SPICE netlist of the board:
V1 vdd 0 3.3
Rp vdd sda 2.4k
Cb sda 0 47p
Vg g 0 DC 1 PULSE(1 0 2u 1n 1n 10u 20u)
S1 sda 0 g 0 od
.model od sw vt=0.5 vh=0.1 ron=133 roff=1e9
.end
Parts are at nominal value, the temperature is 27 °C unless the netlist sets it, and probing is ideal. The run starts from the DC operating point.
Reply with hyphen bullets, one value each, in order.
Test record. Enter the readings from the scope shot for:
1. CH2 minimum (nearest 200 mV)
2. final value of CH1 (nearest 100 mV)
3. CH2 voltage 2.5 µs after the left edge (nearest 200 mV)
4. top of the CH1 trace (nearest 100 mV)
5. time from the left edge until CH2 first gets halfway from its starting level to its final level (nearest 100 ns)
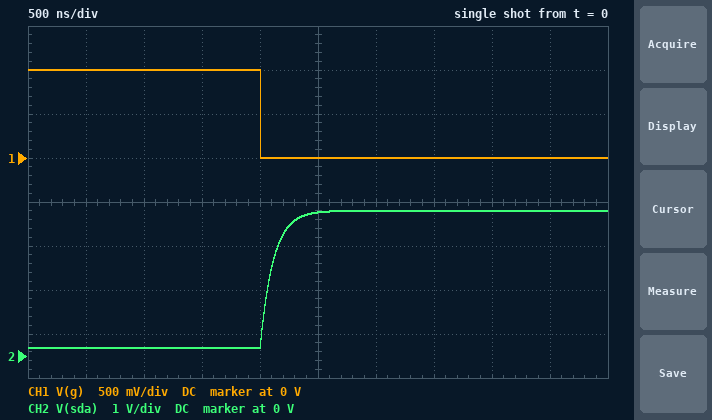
- 200 mV
- 0 V
- 3.2 V
- 1.0 V
- 2.1 µs
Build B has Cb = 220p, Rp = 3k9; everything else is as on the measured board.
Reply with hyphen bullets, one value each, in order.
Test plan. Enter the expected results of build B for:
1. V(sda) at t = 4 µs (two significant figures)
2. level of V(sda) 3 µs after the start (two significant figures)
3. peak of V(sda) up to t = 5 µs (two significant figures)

- 3.0 V
- 2.3 V
- 3.2 V
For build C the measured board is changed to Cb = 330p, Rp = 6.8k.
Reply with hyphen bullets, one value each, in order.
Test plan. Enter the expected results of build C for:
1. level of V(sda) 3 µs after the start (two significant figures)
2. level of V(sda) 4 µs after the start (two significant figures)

- 1.2 V
- 2.0 V
